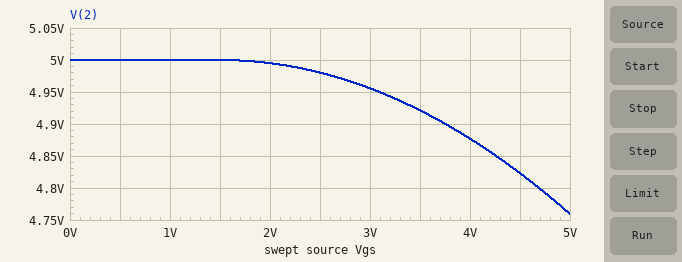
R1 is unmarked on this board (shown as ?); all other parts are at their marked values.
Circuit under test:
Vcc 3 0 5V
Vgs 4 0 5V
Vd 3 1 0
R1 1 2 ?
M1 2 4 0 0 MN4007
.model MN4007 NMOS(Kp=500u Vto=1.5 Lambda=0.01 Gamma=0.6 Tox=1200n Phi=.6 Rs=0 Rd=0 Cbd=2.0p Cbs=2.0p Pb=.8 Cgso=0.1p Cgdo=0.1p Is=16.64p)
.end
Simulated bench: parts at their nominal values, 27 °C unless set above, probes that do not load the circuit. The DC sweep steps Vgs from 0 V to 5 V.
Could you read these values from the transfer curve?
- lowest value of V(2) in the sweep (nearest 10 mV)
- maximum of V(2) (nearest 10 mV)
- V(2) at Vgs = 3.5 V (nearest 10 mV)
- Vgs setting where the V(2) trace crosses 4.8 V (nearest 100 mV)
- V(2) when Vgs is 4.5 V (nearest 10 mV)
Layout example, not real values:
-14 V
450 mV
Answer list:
4.76 V
5.00 V
4.92 V
4.7 V
4.82 V
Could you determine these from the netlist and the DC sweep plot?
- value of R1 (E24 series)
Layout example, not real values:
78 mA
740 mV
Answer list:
75 Ω
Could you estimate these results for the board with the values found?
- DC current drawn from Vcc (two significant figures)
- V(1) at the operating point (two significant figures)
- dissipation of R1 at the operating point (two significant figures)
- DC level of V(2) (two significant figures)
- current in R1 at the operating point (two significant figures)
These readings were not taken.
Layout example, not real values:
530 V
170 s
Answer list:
3.2 mA
5.0 V
770 µW
4.8 V
3.2 mA
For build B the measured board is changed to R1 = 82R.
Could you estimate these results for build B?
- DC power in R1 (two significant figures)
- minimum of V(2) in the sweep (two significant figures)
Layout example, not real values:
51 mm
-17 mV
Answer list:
840 µW
4.7 V
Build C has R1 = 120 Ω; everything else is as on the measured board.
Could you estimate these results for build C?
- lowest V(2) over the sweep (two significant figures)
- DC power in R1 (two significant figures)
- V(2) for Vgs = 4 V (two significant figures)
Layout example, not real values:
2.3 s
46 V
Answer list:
4.6 V
1.2 mW
4.8 V
